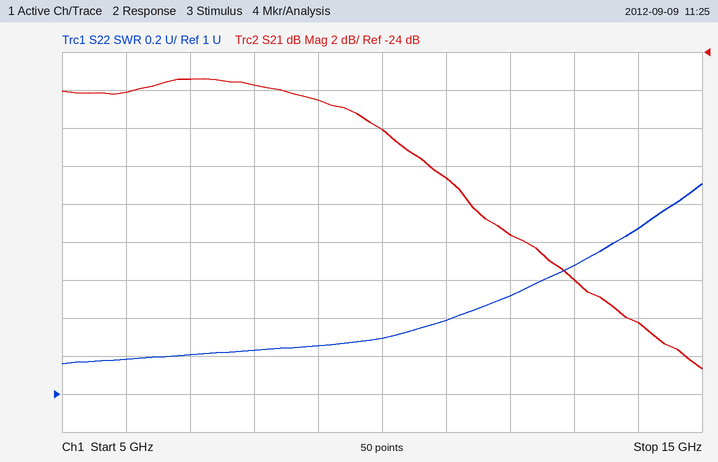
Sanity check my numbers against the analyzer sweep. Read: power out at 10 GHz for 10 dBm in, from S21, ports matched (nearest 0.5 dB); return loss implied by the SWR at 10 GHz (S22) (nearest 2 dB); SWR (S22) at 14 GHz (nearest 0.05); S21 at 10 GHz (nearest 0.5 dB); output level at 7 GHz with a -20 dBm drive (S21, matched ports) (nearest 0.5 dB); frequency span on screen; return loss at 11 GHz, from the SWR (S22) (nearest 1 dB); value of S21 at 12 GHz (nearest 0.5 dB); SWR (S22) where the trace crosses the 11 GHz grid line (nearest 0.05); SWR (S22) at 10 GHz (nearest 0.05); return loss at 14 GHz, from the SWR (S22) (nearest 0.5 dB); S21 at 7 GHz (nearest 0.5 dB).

-18.0 dBm
18 dB
1.85
-28.0 dB
-45.5 dBm
10 GHz
16 dB
-33.5 dB
1.40
1.30
10.5 dB
-25.5 dB
